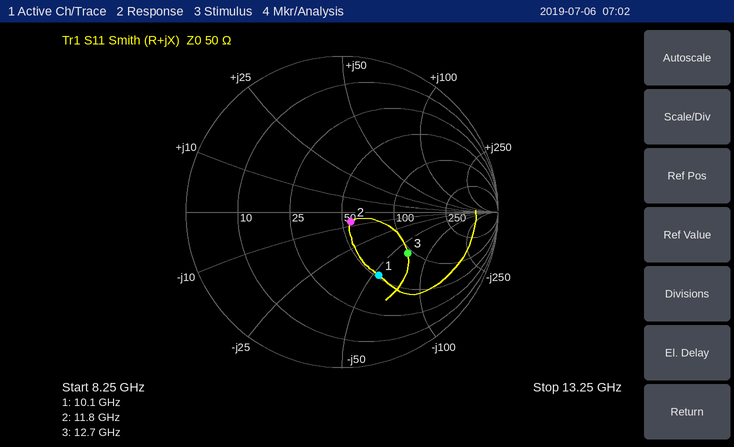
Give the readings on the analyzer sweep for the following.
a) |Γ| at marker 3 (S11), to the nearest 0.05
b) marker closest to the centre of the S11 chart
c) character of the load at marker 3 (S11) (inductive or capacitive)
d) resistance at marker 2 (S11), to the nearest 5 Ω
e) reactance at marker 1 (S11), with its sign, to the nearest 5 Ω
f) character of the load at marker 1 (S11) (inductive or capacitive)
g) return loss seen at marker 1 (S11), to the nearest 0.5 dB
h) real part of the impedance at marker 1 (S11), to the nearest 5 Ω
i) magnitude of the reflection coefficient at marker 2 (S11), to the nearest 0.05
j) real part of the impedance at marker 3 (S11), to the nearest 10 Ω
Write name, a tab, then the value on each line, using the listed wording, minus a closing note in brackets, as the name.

|Γ| at marker 3 (S11), to the nearest 0.05	0.50
marker closest to the centre of the S11 chart	marker 2
character of the load at marker 3 (S11)	capacitive
resistance at marker 2 (S11), to the nearest 5 Ω	55 Ω
reactance at marker 1 (S11), with its sign, to the nearest 5 Ω	-55 Ω
character of the load at marker 1 (S11)	capacitive
return loss seen at marker 1 (S11), to the nearest 0.5 dB	6.5 dB
real part of the impedance at marker 1 (S11), to the nearest 5 Ω	50 Ω
magnitude of the reflection coefficient at marker 2 (S11), to the nearest 0.05	0.10
real part of the impedance at marker 3 (S11), to the nearest 10 Ω	90 Ω
